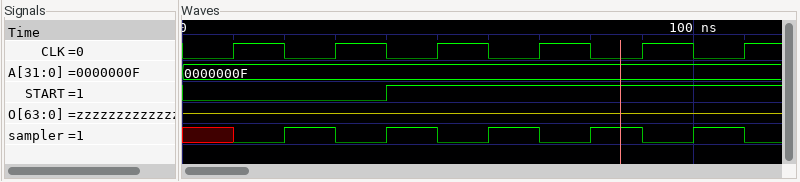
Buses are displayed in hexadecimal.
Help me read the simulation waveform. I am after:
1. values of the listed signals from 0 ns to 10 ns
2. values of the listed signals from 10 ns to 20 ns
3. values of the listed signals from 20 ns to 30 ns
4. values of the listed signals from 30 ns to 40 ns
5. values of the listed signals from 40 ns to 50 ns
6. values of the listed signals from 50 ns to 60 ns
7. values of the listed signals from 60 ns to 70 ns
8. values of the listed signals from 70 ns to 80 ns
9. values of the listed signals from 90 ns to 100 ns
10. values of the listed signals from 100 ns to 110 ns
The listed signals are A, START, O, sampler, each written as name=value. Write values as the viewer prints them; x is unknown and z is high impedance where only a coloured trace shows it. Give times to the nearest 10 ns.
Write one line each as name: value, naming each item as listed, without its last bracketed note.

values of the listed signals from 0 ns to 10 ns: A=0000000F, START=0, O=z, sampler=x
values of the listed signals from 10 ns to 20 ns: A=0000000F, START=0, O=z, sampler=0
values of the listed signals from 20 ns to 30 ns: A=0000000F, START=0, O=z, sampler=1
values of the listed signals from 30 ns to 40 ns: A=0000000F, START=0, O=z, sampler=0
values of the listed signals from 40 ns to 50 ns: A=0000000F, START=1, O=z, sampler=1
values of the listed signals from 50 ns to 60 ns: A=0000000F, START=1, O=z, sampler=0
values of the listed signals from 60 ns to 70 ns: A=0000000F, START=1, O=z, sampler=1
values of the listed signals from 70 ns to 80 ns: A=0000000F, START=1, O=z, sampler=0
values of the listed signals from 90 ns to 100 ns: A=0000000F, START=1, O=z, sampler=0
values of the listed signals from 100 ns to 110 ns: A=0000000F, START=1, O=z, sampler=1
